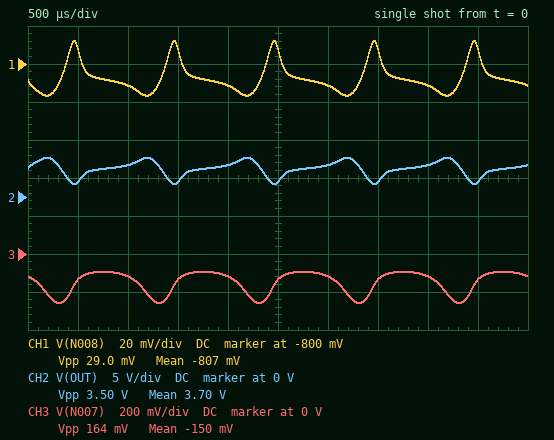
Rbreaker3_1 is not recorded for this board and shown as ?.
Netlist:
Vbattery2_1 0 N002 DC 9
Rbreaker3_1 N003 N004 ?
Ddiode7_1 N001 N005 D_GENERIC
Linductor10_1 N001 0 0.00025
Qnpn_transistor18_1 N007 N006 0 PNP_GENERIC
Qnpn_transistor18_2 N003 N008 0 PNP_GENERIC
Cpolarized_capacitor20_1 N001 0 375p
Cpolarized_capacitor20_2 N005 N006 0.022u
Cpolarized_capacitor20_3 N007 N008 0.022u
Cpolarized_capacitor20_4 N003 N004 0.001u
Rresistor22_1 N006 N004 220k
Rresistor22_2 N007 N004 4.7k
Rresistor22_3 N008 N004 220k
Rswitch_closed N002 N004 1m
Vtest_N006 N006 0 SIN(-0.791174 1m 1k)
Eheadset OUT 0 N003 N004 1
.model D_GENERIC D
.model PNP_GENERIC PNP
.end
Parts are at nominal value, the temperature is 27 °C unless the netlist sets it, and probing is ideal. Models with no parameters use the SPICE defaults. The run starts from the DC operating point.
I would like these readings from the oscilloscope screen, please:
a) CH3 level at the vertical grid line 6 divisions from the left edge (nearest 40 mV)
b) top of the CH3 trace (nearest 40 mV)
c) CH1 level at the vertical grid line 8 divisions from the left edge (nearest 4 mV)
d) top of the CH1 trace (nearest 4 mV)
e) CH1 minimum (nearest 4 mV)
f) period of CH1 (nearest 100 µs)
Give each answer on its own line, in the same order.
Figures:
-120 mV
-80 mV
-812 mV
-788 mV
-816 mV
1.0 ms
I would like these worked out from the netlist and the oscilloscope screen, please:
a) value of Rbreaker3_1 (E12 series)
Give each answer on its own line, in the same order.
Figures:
1 kΩ
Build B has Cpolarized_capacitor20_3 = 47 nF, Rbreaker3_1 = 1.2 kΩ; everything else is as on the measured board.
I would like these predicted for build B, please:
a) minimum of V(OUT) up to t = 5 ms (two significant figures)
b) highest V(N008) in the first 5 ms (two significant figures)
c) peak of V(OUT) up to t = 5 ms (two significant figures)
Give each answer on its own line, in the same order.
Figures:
1.3 V
-780 mV
7.0 V
